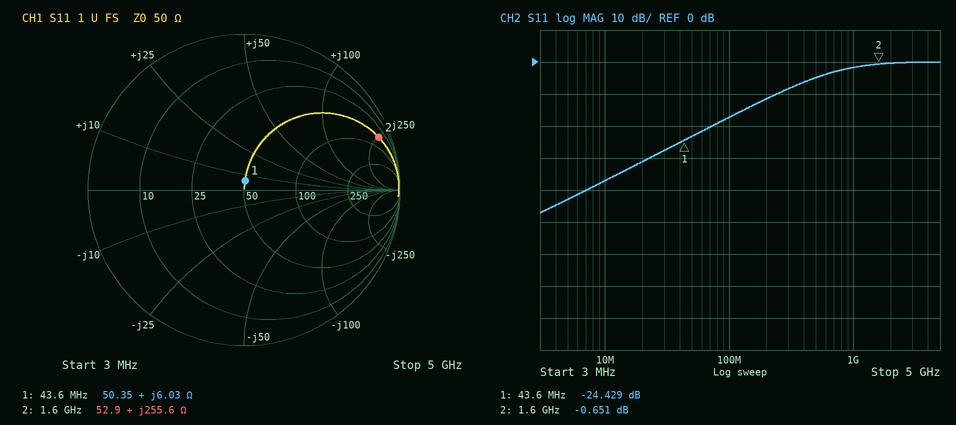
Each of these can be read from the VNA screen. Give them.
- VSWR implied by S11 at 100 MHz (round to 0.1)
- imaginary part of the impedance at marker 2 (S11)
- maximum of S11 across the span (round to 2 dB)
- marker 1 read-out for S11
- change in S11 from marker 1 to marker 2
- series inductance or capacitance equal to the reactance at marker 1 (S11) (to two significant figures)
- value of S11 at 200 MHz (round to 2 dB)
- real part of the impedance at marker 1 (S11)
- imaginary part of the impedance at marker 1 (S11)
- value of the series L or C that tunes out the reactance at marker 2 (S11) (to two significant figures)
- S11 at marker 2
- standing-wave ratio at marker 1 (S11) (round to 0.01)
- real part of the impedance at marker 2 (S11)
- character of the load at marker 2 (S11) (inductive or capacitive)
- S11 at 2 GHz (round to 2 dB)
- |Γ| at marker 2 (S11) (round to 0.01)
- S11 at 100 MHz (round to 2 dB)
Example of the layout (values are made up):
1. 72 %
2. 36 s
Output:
1. 1.3
2. +255.6 Ω
3. 0 dB
4. -24.429 dB
5. 23.778 dB
6. 22 nH
7. -12 dB
8. 50.35 Ω
9. +6.03 Ω
10. 390 fF
11. -0.651 dB
12. 1.13
13. 52.9 Ω
14. inductive
15. 0 dB
16. 0.93
17. -18 dB
